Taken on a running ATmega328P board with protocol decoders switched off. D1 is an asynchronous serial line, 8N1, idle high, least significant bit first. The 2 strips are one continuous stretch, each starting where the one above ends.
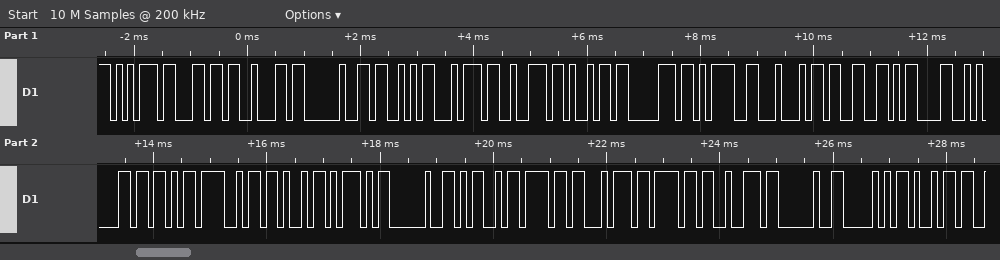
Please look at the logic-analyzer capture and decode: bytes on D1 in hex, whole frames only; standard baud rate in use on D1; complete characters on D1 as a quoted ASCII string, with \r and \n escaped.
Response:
75 6C 62 20 53 74 72 69 70 3D 44 33 0D 0A 5B 4F 4B 5D 20 4D 6F 74 6F 72 20 50 69
9600 baud
"ulb Strip=D3\r\n[OK] Motor Pi"
